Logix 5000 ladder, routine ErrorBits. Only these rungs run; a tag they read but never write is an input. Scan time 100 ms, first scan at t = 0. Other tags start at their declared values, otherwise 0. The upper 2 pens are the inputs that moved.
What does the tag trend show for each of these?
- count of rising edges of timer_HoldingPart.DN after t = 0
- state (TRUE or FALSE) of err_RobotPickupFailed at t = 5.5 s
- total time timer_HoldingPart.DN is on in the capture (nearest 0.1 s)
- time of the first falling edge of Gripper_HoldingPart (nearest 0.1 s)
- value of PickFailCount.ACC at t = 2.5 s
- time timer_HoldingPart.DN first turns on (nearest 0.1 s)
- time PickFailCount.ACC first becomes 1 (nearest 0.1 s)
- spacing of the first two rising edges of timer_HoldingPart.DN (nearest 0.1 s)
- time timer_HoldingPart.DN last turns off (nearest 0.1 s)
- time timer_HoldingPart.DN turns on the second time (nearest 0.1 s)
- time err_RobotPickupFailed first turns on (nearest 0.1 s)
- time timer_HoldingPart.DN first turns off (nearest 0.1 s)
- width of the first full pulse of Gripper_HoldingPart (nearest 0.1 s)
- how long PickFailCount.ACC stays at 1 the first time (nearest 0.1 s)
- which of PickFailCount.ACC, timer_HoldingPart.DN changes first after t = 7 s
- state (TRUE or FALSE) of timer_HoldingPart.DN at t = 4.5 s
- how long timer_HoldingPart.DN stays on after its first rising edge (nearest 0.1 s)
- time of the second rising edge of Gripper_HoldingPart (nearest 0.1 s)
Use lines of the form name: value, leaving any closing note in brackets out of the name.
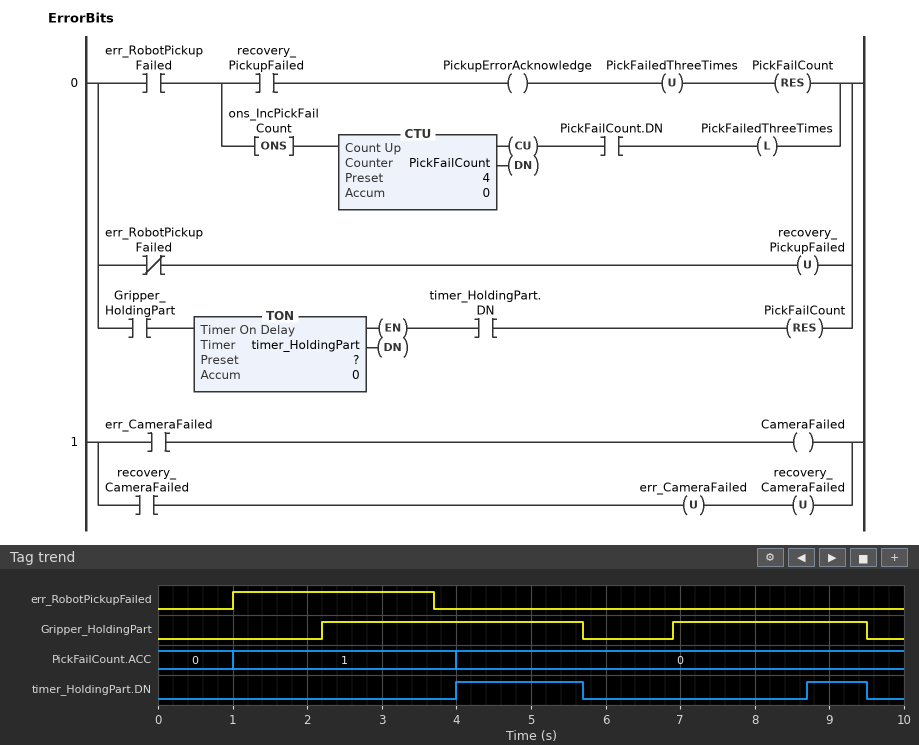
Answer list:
count of rising edges of timer_HoldingPart.DN after t = 0: 2
state (TRUE or FALSE) of err_RobotPickupFailed at t = 5.5 s: FALSE
total time timer_HoldingPart.DN is on in the capture: 2.5 s
time of the first falling edge of Gripper_HoldingPart: 5.7 s
value of PickFailCount.ACC at t = 2.5 s: 1
time timer_HoldingPart.DN first turns on: 4.0 s
time PickFailCount.ACC first becomes 1: 1.0 s
spacing of the first two rising edges of timer_HoldingPart.DN: 4.7 s
time timer_HoldingPart.DN last turns off: 9.5 s
time timer_HoldingPart.DN turns on the second time: 8.7 s
time err_RobotPickupFailed first turns on: 1.0 s
time timer_HoldingPart.DN first turns off: 5.7 s
width of the first full pulse of Gripper_HoldingPart: 3.5 s
how long PickFailCount.ACC stays at 1 the first time: 3.0 s
which of PickFailCount.ACC, timer_HoldingPart.DN changes first after t = 7 s: timer_HoldingPart.DN
state (TRUE or FALSE) of timer_HoldingPart.DN at t = 4.5 s: TRUE
how long timer_HoldingPart.DN stays on after its first rising edge: 1.7 s
time of the second rising edge of Gripper_HoldingPart: 6.9 s
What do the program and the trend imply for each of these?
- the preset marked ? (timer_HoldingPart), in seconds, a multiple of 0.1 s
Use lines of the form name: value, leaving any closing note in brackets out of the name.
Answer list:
the preset marked ? (timer_HoldingPart), in seconds, a multiple of 0.1 s: 1.8 s
